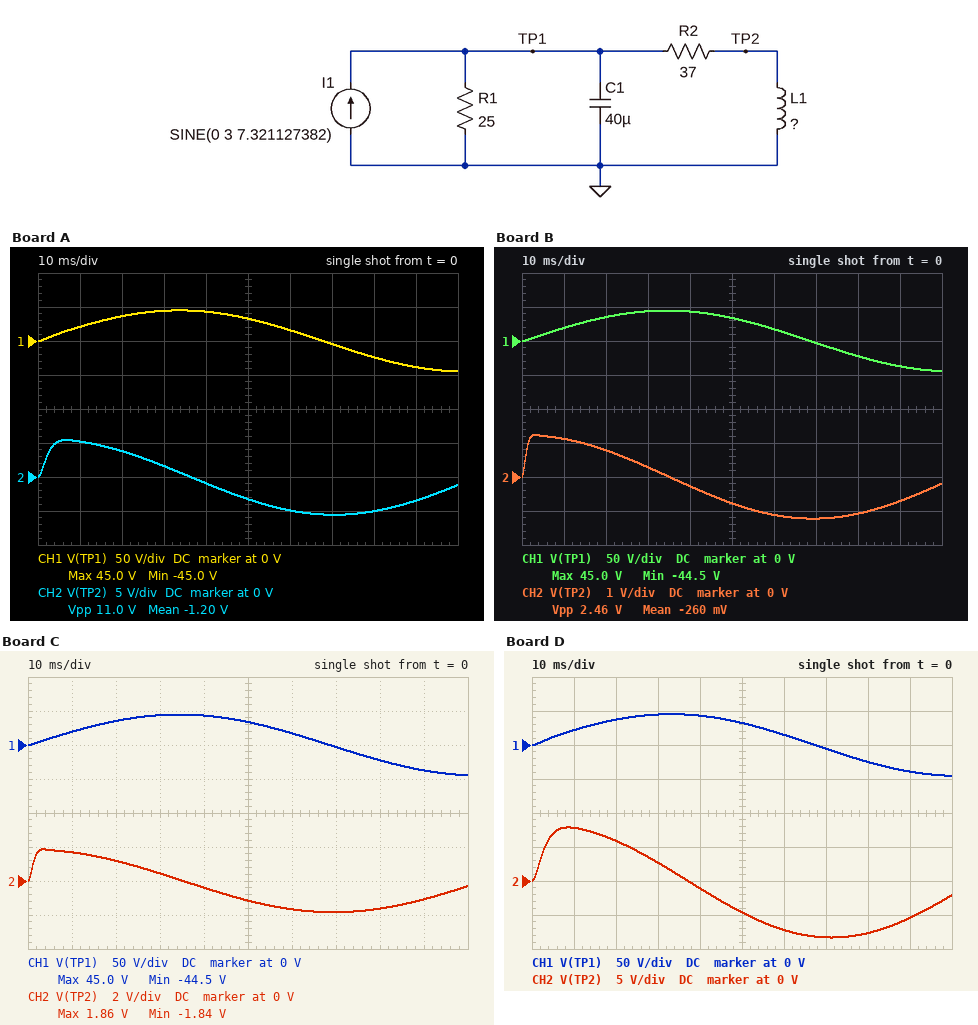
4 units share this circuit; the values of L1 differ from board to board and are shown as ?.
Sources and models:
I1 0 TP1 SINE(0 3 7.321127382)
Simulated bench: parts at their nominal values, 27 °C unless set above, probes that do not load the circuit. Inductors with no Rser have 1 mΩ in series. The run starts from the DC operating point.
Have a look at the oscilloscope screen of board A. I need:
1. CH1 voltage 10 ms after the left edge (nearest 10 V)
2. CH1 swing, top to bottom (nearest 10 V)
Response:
20 V
90 V
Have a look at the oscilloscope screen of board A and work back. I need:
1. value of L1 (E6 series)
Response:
100 mH
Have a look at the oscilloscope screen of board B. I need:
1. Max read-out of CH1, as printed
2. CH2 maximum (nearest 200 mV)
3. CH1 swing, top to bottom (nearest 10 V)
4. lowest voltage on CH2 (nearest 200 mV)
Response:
45.0 V
1.2 V
90 V
-1.2 V
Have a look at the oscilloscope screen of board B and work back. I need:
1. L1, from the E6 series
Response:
22 mH
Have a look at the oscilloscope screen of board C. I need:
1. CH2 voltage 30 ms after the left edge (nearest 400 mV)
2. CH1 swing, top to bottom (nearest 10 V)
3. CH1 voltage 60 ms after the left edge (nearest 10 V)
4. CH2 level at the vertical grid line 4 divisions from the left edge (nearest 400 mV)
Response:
400 mV
90 V
20 V
-400 mV
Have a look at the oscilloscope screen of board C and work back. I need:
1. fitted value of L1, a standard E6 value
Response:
33 mH
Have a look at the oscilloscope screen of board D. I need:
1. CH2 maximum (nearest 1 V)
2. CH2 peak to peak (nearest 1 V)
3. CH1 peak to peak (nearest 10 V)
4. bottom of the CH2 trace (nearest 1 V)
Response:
8 V
16 V
90 V
-8 V
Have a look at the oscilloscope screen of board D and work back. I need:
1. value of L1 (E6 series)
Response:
150 mH
